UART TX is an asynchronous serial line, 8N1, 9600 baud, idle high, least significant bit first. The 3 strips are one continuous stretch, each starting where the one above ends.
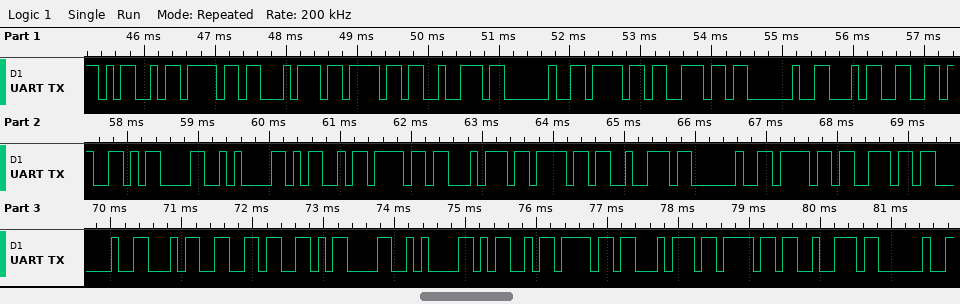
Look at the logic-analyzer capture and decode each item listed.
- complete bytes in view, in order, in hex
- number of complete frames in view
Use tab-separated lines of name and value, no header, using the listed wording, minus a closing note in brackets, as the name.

complete bytes in view, in order, in hex	4D 6F 74 6F 72 20 6F 6E 20 34 36 0D 0A 4D 6F 74 6F 72 20 6F 6E 20 34 36 0D 0A 4D 6F 74 6F 72 20
number of complete frames in view	32
